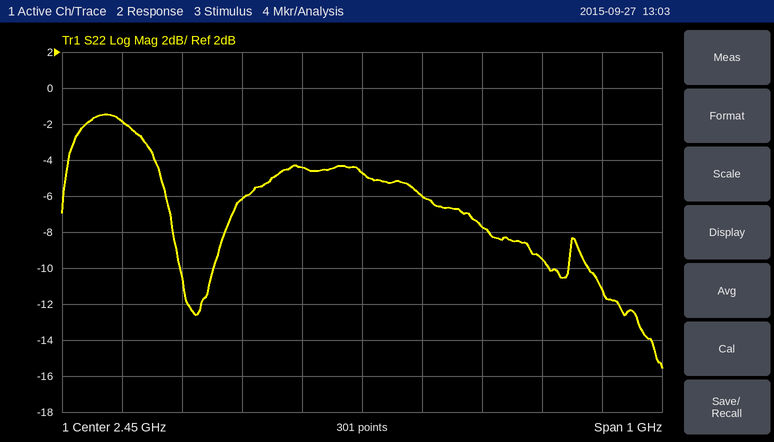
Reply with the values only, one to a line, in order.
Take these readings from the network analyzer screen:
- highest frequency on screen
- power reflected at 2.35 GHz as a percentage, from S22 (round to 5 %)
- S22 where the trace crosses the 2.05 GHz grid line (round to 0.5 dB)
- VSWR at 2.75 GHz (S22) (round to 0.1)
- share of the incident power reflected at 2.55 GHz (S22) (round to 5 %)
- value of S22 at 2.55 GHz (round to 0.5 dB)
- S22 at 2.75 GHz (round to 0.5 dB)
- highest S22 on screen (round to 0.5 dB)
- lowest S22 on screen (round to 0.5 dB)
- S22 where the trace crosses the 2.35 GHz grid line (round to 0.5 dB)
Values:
2.95 GHz
35 %
-2.0 dB
2.0
25 %
-6.0 dB
-9.5 dB
-1.5 dB
-15.5 dB
-4.5 dB
